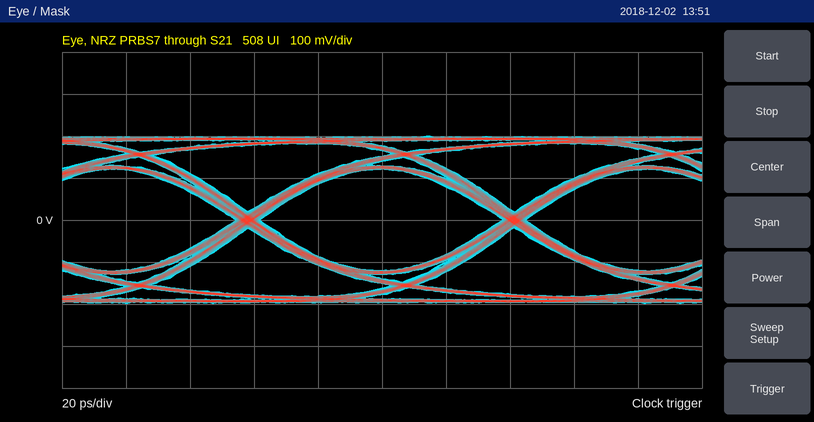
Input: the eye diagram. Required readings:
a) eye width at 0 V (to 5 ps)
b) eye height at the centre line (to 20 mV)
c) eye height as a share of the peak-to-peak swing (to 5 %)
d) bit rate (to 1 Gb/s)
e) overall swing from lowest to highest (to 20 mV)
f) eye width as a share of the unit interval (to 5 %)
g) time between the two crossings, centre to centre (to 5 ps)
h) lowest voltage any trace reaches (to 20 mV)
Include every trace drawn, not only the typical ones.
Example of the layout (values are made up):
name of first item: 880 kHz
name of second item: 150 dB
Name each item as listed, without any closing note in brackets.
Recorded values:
eye width at 0 V: 75 ps
eye height at the centre line: 240 mV
eye height as a share of the peak-to-peak swing: 60 %
bit rate: 12 Gb/s
overall swing from lowest to highest: 400 mV
eye width as a share of the unit interval: 90 %
time between the two crossings, centre to centre: 85 ps
lowest voltage any trace reaches: -200 mV
